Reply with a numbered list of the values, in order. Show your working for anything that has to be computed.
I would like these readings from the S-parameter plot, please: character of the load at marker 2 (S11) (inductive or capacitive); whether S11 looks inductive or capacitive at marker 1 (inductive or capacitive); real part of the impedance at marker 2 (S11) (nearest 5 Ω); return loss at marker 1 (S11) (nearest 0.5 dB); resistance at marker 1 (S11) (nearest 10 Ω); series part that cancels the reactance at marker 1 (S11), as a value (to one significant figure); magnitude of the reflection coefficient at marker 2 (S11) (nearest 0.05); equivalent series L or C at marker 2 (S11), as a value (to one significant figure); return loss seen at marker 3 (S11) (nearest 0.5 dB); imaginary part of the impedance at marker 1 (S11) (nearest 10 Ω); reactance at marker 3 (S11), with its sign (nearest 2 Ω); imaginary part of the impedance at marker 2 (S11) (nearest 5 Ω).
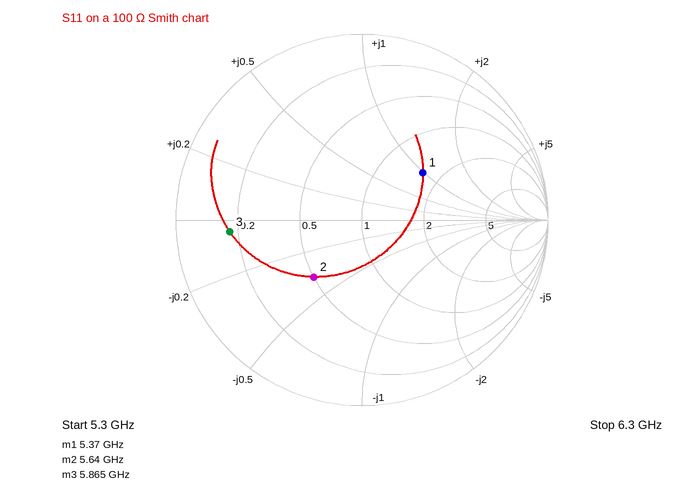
1. capacitive
2. inductive
3. 50 Ω
4. 7.5 dB
5. 160 Ω
6. C = 1/(2π × 5.37 GHz × 100 Ω) ≈ 296 fF, so 300 fF to one significant figure
7. 0.40
8. C = 1/(2π × 5.64 GHz × 35 Ω) ≈ 806 fF, so 800 fF to one significant figure
9. 3.0 dB
10. +100 Ω
11. -4 Ω
12. -35 Ω
